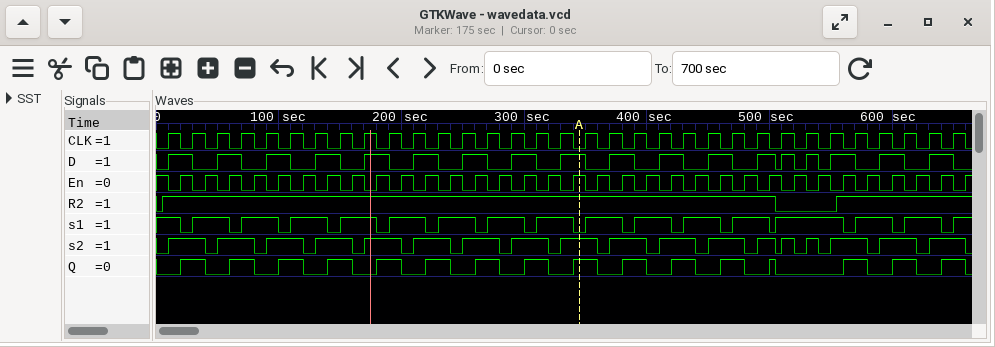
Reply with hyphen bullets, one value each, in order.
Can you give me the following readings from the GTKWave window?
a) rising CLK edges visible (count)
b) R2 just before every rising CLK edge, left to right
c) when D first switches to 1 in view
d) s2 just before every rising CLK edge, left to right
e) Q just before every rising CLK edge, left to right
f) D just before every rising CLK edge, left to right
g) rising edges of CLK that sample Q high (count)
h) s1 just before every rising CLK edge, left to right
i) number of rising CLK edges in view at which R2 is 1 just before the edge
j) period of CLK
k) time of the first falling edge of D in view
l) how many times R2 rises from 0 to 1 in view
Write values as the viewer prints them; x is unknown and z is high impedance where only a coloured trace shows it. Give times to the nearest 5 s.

- 33
- 1 1 1 1 1 1 1 1 1 1 1 1 1 1 1 1 1 1 1 1 1 1 1 1 1 0 0 0 1 1 1 1 1
- 10 s
- 0 1 0 1 0 1 0 1 0 1 0 1 0 1 0 1 0 1 0 1 0 1 0 1 0 0 0 0 1 0 1 0 1
- 0 1 0 1 0 1 0 1 0 1 0 1 0 1 0 1 0 1 0 1 0 1 0 1 0 0 0 0 1 0 1 0 1
- 0 1 0 1 0 1 0 1 0 1 0 1 0 1 0 1 0 1 0 1 0 1 0 1 0 0 0 0 1 0 1 0 1
- 15
- 1 0 1 0 1 0 1 0 1 0 1 0 1 0 1 0 1 0 1 0 1 0 1 0 1 1 1 1 0 1 0 1 0
- 30
- 20 s
- 30 s
- 2
